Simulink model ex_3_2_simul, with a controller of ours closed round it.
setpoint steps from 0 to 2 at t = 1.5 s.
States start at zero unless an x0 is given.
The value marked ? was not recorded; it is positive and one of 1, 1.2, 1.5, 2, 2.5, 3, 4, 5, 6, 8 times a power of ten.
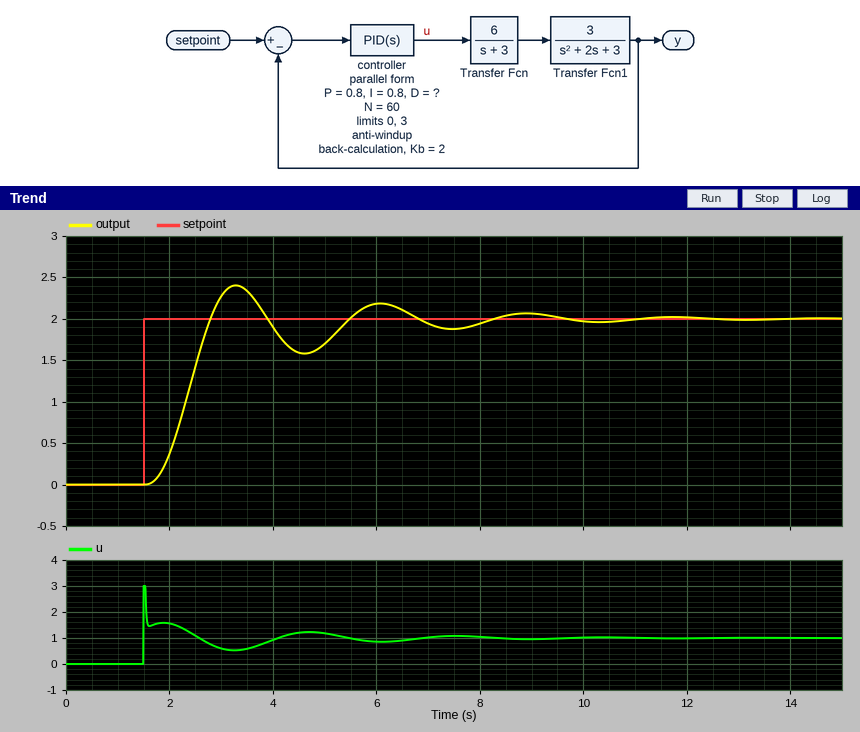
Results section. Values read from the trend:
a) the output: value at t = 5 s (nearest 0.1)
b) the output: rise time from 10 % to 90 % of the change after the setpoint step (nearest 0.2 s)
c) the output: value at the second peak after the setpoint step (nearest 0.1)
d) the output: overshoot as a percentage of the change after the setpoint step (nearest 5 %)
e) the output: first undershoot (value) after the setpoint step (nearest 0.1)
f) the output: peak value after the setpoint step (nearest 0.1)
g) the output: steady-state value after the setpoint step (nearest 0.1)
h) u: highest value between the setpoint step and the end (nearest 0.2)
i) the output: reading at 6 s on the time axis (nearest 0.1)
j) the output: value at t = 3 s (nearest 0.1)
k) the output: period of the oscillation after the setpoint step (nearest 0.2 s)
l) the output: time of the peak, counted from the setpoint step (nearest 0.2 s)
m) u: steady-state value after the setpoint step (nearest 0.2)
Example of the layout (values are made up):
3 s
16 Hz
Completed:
1.7
0.8 s
2.2
20 %
1.6
2.4
2.0
3.0
2.2
2.3
2.8 s
1.8 s
1.0
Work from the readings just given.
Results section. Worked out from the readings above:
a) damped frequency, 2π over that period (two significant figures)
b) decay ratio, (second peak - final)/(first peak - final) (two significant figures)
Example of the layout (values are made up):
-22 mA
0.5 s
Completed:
2.2 rad/s
0.50
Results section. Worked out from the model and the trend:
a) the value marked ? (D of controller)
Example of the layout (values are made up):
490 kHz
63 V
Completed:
0.12
